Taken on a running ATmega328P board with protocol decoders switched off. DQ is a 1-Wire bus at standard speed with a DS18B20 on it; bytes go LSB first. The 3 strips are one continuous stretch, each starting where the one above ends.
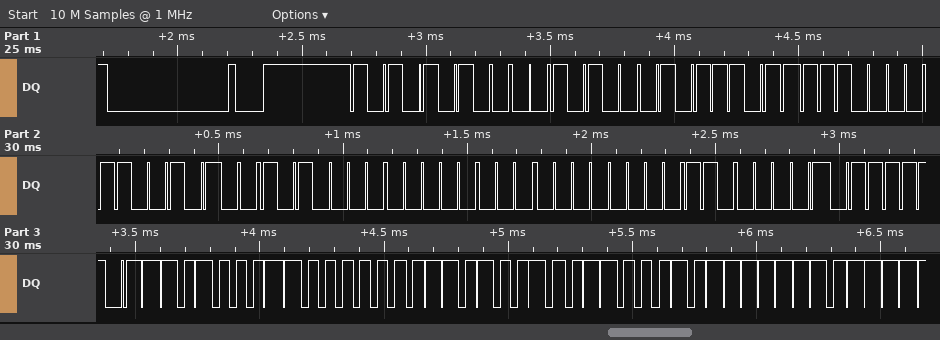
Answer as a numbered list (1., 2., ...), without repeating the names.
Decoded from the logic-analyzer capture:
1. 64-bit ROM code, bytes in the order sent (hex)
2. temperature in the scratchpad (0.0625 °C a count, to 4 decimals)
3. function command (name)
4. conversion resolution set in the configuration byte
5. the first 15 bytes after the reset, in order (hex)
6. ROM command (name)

1. 28 BA 0F 53 0A 00 00 83
2. 24.6875 °C
3. Read Scratchpad
4. 12 bits
5. 55 28 BA 0F 53 0A 00 00 83 BE 8B 01 4B 46 7F
6. Match ROM
